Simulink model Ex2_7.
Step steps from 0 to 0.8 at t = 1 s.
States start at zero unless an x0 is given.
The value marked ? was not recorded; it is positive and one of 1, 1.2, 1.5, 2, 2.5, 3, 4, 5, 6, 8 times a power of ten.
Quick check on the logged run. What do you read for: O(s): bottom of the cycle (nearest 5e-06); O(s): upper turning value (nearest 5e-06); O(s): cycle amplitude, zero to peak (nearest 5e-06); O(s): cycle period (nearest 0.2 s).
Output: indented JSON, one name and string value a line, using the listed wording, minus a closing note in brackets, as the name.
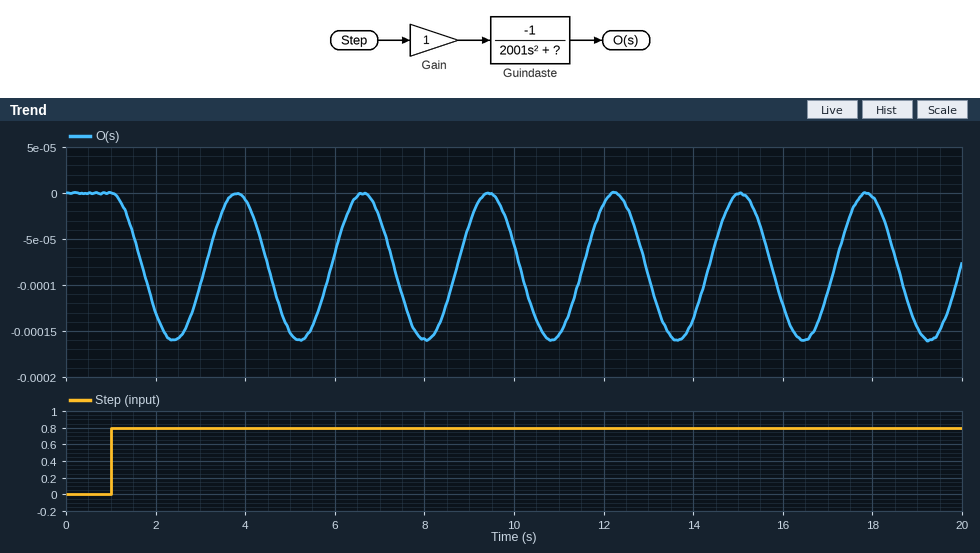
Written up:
{
  "O(s): bottom of the cycle": "-0.000160",
  "O(s): upper turning value": "0.000000",
  "O(s): cycle amplitude, zero to peak": "0.000080",
  "O(s): cycle period": "2.8 s"
}
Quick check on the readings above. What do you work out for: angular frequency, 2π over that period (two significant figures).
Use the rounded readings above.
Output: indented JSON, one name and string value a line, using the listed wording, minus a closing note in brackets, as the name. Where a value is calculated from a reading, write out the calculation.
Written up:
{
  "angular frequency, 2π over that period": "2π / 2.8 = 2.2 rad/s"
}
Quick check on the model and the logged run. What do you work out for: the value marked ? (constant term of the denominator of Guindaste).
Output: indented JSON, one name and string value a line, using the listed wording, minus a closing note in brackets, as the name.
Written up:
{
  "the value marked ?": "10000"
}
